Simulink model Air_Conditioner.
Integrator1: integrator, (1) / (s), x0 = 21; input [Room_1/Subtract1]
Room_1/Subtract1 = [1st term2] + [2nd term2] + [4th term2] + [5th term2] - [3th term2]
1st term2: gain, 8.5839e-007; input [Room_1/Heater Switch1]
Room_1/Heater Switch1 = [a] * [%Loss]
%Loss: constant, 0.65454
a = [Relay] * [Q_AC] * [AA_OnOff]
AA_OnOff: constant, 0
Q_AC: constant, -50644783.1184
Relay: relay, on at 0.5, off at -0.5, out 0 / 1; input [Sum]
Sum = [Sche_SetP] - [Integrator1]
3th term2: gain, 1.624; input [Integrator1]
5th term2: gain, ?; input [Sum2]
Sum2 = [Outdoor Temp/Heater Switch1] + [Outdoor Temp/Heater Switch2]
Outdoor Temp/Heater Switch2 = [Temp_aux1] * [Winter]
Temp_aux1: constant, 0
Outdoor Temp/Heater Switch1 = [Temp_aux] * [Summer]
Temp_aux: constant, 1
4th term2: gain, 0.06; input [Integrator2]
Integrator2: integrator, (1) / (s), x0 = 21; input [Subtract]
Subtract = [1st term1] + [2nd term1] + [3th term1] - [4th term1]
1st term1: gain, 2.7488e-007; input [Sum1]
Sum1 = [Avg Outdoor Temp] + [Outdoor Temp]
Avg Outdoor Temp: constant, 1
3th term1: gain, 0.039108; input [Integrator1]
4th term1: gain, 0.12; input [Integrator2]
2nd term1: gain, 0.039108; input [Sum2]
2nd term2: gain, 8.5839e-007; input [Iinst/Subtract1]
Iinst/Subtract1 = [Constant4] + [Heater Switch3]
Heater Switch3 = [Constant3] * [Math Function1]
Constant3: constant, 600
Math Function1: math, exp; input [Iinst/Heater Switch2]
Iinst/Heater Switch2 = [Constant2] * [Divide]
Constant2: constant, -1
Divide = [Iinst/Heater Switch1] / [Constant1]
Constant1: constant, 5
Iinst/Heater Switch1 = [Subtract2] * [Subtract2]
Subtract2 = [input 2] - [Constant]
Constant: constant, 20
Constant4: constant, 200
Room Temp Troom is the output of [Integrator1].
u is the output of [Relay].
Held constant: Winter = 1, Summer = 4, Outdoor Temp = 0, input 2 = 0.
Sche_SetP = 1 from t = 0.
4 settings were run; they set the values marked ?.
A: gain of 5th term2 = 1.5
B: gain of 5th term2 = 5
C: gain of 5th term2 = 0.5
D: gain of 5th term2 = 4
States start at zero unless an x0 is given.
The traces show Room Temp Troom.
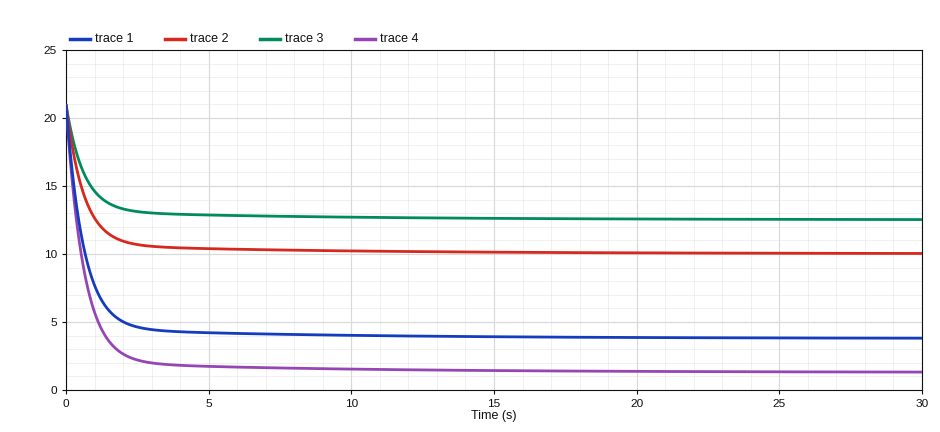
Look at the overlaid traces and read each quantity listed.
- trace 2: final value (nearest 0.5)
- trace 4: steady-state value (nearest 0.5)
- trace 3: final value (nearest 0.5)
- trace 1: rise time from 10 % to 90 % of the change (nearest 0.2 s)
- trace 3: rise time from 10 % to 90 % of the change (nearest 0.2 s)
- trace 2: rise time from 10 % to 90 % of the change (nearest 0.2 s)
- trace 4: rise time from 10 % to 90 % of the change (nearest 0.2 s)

10.0
1.5
12.5
1.6 s
1.8 s
1.8 s
1.6 s
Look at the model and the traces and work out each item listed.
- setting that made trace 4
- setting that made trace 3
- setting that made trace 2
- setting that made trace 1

C
B
D
A
